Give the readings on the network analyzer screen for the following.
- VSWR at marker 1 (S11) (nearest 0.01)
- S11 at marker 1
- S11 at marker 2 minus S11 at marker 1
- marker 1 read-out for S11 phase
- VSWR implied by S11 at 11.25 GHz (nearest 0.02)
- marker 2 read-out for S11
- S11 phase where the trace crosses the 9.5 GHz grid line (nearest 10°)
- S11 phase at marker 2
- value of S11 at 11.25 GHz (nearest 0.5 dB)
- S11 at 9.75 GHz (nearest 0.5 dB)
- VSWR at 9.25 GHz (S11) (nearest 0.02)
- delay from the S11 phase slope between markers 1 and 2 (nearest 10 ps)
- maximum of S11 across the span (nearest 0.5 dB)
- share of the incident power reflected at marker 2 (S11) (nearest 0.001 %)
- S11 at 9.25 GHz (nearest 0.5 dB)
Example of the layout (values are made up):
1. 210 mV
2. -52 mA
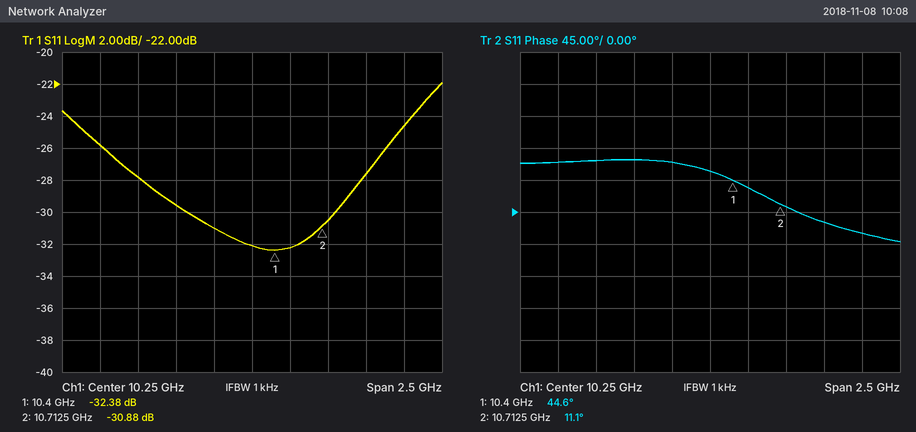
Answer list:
1. 1.05
2. -32.38 dB
3. 1.50 dB
4. 44.6°
5. 1.12
6. -30.88 dB
7. 70°
8. 11.1°
9. -24.5 dB
10. -29.5 dB
11. 1.10
12. 300 ps
13. -22.0 dB
14. 0.082 %
15. -26.0 dB
